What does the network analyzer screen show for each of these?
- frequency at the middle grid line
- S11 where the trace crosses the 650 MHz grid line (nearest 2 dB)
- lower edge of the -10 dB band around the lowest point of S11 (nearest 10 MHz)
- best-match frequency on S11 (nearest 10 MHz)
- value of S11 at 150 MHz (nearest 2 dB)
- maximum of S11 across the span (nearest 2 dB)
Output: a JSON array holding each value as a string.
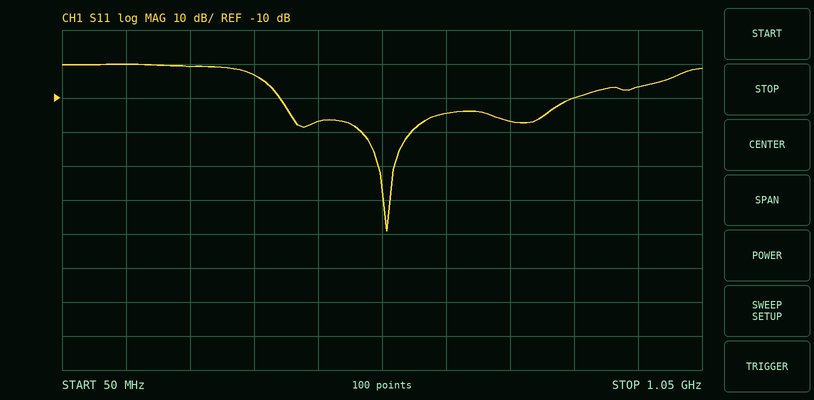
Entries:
["550 MHz", "-14 dB", "390 MHz", "560 MHz", "0 dB", "0 dB"]
